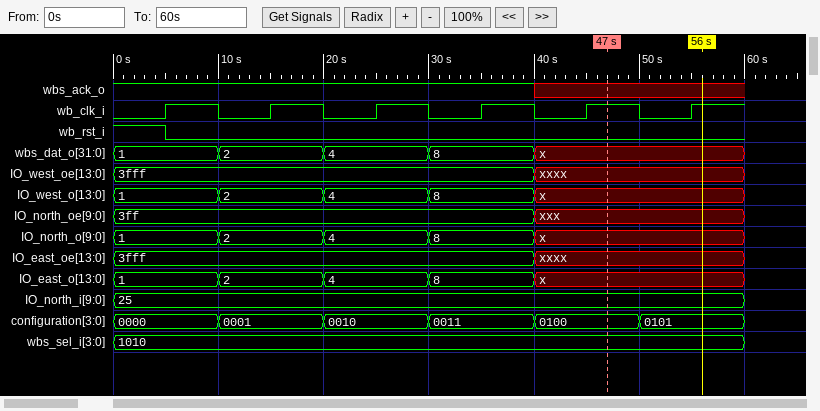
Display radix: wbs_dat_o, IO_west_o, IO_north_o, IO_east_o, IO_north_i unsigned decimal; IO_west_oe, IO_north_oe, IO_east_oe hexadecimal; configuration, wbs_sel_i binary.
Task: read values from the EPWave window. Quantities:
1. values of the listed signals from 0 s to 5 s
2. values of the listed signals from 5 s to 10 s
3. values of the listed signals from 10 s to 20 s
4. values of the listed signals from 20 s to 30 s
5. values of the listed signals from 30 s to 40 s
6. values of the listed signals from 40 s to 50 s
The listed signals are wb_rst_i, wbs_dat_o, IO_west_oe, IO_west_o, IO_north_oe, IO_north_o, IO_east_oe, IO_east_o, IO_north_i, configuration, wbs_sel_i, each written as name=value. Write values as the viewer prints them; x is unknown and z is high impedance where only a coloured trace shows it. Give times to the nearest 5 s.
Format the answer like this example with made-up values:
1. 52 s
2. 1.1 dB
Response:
1. wb_rst_i=1, wbs_dat_o=1, IO_west_oe=3fff, IO_west_o=1, IO_north_oe=3ff, IO_north_o=1, IO_east_oe=3fff, IO_east_o=1, IO_north_i=25, configuration=0000, wbs_sel_i=1010
2. wb_rst_i=0, wbs_dat_o=1, IO_west_oe=3fff, IO_west_o=1, IO_north_oe=3ff, IO_north_o=1, IO_east_oe=3fff, IO_east_o=1, IO_north_i=25, configuration=0000, wbs_sel_i=1010
3. wb_rst_i=0, wbs_dat_o=2, IO_west_oe=3fff, IO_west_o=2, IO_north_oe=3ff, IO_north_o=2, IO_east_oe=3fff, IO_east_o=2, IO_north_i=25, configuration=0001, wbs_sel_i=1010
4. wb_rst_i=0, wbs_dat_o=4, IO_west_oe=3fff, IO_west_o=4, IO_north_oe=3ff, IO_north_o=4, IO_east_oe=3fff, IO_east_o=4, IO_north_i=25, configuration=0010, wbs_sel_i=1010
5. wb_rst_i=0, wbs_dat_o=8, IO_west_oe=3fff, IO_west_o=8, IO_north_oe=3ff, IO_north_o=8, IO_east_oe=3fff, IO_east_o=8, IO_north_i=25, configuration=0011, wbs_sel_i=1010
6. wb_rst_i=0, wbs_dat_o=x, IO_west_oe=xxxx, IO_west_o=x, IO_north_oe=xxx, IO_north_o=x, IO_east_oe=xxxx, IO_east_o=x, IO_north_i=25, configuration=0100, wbs_sel_i=1010
